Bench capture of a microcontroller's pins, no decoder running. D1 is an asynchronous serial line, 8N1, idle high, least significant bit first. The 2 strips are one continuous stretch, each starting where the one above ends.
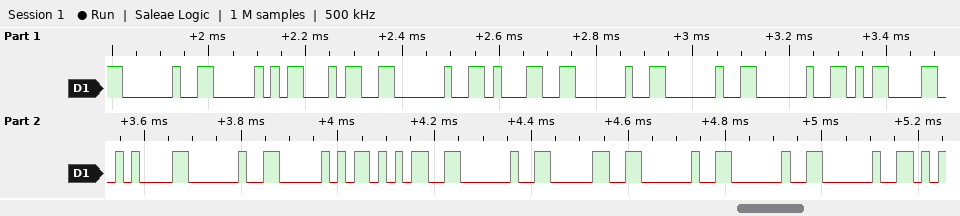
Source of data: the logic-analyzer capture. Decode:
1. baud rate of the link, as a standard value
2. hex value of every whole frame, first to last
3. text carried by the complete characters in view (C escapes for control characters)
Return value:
57600 baud
20 50 34 20 31 20 20 20 0D 0A 20 50 35 20 30 20 20 20
" P4 1   \r\n P5 0   "
